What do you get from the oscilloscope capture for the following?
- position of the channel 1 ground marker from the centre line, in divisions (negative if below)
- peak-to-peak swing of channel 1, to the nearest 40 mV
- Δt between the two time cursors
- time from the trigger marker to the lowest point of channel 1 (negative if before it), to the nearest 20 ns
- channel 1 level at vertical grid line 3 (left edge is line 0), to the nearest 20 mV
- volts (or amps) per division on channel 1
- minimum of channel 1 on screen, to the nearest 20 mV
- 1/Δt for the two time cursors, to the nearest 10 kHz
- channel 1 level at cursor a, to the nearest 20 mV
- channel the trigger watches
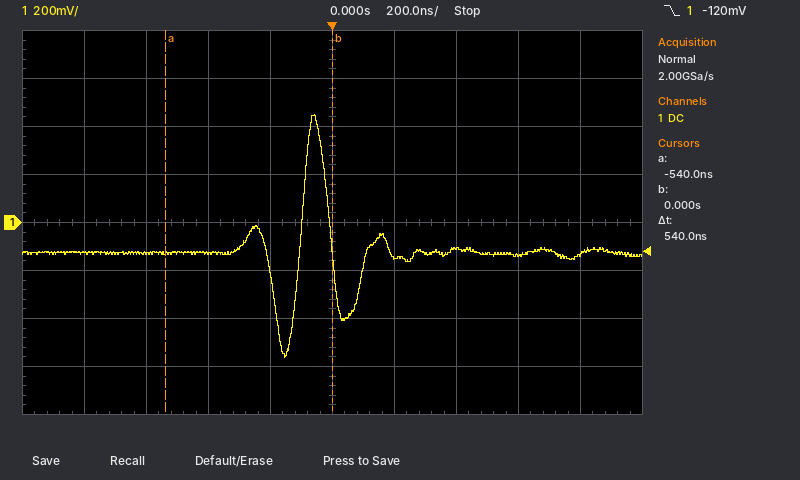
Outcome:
0.0 div
1.00 V
540 ns
-160 ns
-120 mV
200 mV
-560 mV
1.85 MHz
-120 mV
channel 1
